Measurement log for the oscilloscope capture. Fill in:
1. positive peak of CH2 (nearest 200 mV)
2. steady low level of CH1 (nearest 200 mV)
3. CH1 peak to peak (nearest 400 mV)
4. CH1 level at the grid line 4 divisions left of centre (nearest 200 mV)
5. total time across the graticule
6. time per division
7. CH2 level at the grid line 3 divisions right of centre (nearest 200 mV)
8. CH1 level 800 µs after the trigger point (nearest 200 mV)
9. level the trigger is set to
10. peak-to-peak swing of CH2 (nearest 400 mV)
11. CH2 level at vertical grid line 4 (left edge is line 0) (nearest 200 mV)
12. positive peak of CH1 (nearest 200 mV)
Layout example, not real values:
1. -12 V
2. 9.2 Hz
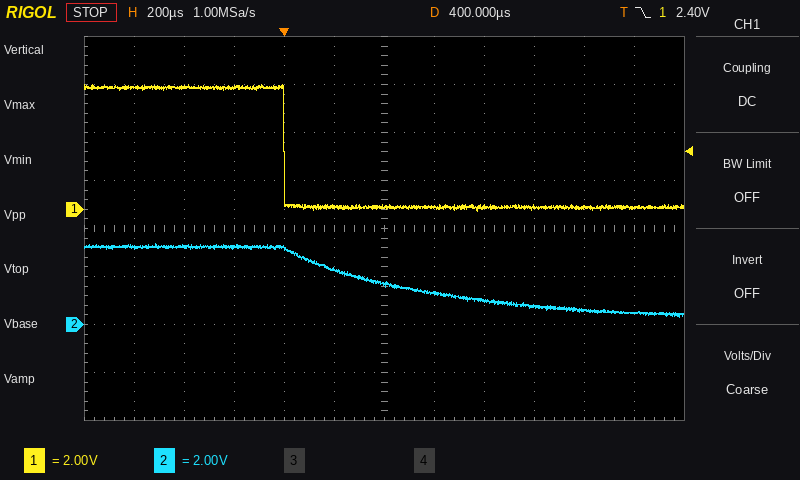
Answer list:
1. 3.4 V
2. 0.0 V
3. 5.2 V
4. 5.0 V
5. 2.4 ms
6. 200 µs
7. 800 mV
8. 0.0 V
9. 2.40 V
10. 3.2 V
11. 3.2 V
12. 5.2 V
